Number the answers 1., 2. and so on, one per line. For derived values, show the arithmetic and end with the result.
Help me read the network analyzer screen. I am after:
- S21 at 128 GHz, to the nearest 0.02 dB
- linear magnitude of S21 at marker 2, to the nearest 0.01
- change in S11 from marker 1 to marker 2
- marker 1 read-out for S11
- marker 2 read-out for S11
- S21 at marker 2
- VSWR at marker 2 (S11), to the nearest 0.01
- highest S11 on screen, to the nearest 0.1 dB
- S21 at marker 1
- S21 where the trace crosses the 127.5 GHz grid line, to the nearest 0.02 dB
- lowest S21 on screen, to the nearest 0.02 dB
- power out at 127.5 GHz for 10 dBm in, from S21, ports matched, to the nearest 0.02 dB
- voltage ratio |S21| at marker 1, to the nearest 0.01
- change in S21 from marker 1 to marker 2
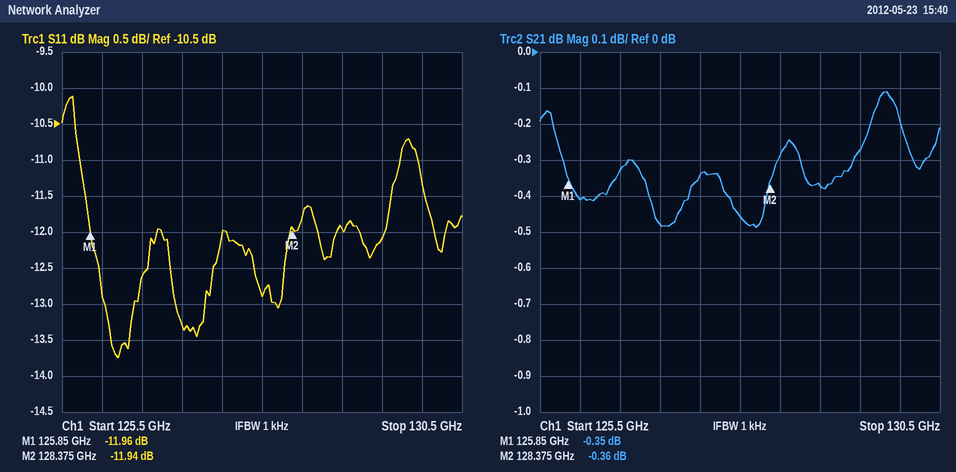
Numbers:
1. -0.46 dB
2. 10^(-0.36/20) ≈ 0.96
3. -11.94 − (-11.96) = 0.02 dB
4. -11.96 dB
5. -11.94 dB
6. -0.36 dB
7. (1 + 0.2529)/(1 − 0.2529) ≈ 1.68
8. -10.1 dB
9. -0.35 dB
10. -0.34 dB
11. -0.48 dB
12. 10 dBm + (-0.34 dB) = 9.66 dBm
13. 10^(-0.35/20) ≈ 0.96
14. -0.36 − (-0.35) = -0.01 dB
